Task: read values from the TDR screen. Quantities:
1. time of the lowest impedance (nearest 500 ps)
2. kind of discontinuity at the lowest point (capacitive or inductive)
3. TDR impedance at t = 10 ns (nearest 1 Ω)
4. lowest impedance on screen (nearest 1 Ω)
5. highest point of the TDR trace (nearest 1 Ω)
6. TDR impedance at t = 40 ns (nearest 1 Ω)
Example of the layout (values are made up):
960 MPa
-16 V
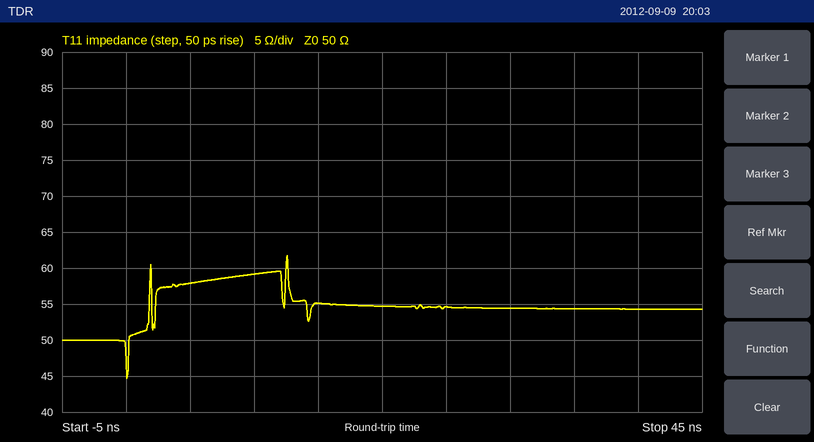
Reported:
0.0 ns
capacitive
59 Ω
45 Ω
62 Ω
54 Ω
